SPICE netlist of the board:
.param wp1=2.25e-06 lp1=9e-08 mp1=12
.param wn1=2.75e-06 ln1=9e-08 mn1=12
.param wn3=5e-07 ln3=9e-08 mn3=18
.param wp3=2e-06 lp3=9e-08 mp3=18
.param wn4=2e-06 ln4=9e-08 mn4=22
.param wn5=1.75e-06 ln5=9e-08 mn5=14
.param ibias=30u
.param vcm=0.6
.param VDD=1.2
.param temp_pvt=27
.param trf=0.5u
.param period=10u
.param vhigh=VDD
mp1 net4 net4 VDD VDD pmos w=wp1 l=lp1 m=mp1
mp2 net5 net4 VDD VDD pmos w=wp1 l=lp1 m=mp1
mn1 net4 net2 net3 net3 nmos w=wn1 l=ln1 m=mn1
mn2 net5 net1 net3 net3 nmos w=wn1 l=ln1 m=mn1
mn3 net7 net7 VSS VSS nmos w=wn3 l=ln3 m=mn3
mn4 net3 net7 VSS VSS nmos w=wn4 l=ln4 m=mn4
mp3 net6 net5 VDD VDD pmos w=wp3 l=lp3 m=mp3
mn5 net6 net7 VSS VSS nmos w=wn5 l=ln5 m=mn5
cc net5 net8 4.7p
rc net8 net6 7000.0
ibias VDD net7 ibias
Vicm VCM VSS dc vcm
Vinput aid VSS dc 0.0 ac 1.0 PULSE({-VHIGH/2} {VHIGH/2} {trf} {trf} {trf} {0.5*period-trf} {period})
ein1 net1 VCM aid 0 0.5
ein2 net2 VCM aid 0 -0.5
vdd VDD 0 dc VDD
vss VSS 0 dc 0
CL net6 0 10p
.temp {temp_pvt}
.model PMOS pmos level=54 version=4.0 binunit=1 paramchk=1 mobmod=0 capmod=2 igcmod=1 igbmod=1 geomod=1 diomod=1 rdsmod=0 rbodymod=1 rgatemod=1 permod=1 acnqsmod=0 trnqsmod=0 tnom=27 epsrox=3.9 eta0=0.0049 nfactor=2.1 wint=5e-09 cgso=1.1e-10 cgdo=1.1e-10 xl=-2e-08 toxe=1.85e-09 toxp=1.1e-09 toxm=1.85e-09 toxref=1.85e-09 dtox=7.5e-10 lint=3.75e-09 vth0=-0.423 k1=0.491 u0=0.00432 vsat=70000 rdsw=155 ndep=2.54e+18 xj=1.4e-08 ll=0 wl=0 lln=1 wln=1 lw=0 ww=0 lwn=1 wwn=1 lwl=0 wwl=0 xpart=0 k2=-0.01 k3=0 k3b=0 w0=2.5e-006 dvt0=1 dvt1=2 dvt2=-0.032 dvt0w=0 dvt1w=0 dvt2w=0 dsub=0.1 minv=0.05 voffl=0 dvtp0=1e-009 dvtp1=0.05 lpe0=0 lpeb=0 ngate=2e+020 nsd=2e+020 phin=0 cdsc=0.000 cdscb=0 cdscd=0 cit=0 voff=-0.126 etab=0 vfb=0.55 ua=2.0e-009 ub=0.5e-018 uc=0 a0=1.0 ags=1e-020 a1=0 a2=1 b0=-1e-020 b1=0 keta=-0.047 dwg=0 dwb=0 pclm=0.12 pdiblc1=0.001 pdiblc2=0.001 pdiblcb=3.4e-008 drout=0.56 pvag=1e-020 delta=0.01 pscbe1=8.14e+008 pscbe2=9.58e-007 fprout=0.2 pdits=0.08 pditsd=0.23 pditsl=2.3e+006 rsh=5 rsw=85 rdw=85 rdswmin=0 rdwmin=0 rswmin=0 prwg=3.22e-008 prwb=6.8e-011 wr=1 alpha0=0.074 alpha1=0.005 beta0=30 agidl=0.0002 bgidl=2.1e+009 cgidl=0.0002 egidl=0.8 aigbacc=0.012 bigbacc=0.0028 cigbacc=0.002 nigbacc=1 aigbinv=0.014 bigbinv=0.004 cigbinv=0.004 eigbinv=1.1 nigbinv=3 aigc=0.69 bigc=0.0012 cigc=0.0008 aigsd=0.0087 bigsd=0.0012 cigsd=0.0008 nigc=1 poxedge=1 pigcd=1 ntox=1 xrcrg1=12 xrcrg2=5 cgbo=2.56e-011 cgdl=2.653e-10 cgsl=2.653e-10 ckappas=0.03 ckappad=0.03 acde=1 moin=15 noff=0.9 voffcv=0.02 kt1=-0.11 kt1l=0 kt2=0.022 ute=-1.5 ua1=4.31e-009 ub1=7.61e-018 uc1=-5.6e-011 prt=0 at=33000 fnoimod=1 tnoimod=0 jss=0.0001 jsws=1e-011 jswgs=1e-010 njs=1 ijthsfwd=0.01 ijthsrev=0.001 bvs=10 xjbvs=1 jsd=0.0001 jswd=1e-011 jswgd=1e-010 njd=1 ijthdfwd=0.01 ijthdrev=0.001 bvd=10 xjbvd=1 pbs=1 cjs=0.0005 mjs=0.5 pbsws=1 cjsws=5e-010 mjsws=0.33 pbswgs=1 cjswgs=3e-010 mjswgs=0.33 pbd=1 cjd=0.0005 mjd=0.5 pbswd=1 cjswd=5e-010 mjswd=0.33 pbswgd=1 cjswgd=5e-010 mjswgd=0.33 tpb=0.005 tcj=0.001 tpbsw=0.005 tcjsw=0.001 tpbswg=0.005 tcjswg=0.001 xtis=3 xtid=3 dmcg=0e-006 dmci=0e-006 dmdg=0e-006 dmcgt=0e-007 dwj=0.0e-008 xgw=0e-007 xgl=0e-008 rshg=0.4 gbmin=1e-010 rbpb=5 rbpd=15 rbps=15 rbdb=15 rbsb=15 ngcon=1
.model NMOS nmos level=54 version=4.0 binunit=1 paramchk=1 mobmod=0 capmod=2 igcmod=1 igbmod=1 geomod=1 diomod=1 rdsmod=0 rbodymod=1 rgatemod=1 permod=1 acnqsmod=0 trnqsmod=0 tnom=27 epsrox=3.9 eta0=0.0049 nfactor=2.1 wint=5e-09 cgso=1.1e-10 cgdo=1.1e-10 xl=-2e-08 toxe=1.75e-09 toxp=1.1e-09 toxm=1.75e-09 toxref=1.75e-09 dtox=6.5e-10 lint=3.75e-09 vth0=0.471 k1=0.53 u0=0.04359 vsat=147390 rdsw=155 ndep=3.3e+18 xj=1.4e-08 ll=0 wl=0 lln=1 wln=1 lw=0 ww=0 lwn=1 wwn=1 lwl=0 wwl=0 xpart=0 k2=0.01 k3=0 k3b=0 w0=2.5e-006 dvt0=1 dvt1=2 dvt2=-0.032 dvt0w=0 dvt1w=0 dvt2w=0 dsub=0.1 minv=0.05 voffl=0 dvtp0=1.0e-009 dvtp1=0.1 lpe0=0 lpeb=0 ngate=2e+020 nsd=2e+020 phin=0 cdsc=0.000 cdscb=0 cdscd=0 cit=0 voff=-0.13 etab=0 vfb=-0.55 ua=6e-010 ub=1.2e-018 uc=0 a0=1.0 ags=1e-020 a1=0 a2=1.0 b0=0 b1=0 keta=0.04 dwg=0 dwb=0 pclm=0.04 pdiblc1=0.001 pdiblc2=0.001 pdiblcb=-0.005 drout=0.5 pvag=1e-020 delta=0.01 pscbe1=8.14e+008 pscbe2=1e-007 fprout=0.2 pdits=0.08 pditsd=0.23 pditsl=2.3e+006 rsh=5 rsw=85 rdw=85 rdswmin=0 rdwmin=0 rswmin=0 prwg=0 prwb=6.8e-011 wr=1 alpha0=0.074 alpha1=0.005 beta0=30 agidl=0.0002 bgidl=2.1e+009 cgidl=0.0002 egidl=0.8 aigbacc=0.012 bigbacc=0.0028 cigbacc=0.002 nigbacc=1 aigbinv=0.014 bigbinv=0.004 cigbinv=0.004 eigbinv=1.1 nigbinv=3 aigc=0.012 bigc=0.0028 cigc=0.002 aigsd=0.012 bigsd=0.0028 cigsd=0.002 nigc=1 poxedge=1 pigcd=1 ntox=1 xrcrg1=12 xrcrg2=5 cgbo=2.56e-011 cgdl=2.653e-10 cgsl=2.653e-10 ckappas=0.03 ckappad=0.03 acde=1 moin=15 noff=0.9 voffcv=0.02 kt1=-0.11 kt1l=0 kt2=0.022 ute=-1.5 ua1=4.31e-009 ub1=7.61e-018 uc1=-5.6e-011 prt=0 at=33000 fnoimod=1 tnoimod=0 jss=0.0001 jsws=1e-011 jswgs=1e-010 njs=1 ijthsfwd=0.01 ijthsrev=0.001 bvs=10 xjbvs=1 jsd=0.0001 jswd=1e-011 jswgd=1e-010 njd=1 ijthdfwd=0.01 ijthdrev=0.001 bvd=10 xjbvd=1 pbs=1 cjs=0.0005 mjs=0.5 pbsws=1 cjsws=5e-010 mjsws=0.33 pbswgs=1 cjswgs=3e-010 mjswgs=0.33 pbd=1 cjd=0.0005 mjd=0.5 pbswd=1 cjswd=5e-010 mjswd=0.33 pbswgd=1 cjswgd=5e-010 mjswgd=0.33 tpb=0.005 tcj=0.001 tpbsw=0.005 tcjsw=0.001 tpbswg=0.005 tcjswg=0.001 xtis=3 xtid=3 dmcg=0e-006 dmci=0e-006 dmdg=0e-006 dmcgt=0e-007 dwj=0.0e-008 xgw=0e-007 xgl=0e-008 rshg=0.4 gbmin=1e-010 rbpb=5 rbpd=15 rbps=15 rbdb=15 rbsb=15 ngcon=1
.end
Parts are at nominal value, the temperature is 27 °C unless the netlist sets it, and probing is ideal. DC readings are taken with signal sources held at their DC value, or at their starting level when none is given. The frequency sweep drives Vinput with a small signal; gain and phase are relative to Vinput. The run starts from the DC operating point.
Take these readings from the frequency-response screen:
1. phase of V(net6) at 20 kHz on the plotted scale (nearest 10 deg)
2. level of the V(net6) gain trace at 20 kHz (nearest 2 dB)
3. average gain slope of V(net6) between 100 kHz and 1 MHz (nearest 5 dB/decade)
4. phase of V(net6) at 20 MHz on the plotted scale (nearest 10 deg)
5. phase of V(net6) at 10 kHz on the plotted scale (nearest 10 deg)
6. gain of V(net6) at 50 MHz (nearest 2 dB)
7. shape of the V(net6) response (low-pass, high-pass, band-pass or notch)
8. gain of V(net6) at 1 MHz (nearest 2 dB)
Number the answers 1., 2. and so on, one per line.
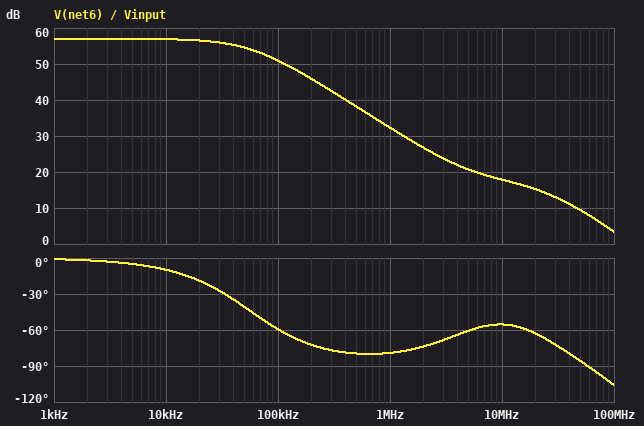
1. -20 deg
2. 56 dB
3. -20 dB/decade
4. -60 deg
5. -10 deg
6. 10 dB
7. low-pass
8. 32 dB
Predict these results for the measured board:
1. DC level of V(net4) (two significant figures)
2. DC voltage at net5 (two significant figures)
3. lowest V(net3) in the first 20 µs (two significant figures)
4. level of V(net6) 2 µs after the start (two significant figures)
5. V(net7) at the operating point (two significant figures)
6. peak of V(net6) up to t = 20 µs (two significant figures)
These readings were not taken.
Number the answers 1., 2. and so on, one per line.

1. 730 mV
2. 730 mV
3. 9.9 mV
4. 1.2 V
5. 390 mV
6. 1.2 V
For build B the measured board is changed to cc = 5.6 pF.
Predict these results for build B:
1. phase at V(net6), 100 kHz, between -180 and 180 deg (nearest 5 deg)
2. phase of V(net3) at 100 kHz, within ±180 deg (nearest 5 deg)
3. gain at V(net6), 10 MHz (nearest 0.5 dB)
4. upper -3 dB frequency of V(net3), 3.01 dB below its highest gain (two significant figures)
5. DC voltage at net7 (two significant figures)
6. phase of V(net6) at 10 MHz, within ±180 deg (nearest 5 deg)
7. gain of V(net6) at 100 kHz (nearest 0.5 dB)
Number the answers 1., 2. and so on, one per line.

1. -65 deg
2. 125 deg
3. 17.5 dB
4. 49 kHz
5. 390 mV
6. -50 deg
7. 50.0 dB
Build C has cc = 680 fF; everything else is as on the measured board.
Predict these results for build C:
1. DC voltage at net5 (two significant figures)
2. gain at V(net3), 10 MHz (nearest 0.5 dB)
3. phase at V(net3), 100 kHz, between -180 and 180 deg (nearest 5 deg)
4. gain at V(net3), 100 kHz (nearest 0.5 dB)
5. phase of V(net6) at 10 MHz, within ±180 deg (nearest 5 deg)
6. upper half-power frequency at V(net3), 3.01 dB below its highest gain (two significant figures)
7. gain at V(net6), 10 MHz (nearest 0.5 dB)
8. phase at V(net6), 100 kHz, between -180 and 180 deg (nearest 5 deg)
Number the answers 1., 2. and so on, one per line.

1. 730 mV
2. -21.5 dB
3. 170 deg
4. -12.5 dB
5. -95 deg
6. 340 kHz
7. 26.0 dB
8. -20 deg
